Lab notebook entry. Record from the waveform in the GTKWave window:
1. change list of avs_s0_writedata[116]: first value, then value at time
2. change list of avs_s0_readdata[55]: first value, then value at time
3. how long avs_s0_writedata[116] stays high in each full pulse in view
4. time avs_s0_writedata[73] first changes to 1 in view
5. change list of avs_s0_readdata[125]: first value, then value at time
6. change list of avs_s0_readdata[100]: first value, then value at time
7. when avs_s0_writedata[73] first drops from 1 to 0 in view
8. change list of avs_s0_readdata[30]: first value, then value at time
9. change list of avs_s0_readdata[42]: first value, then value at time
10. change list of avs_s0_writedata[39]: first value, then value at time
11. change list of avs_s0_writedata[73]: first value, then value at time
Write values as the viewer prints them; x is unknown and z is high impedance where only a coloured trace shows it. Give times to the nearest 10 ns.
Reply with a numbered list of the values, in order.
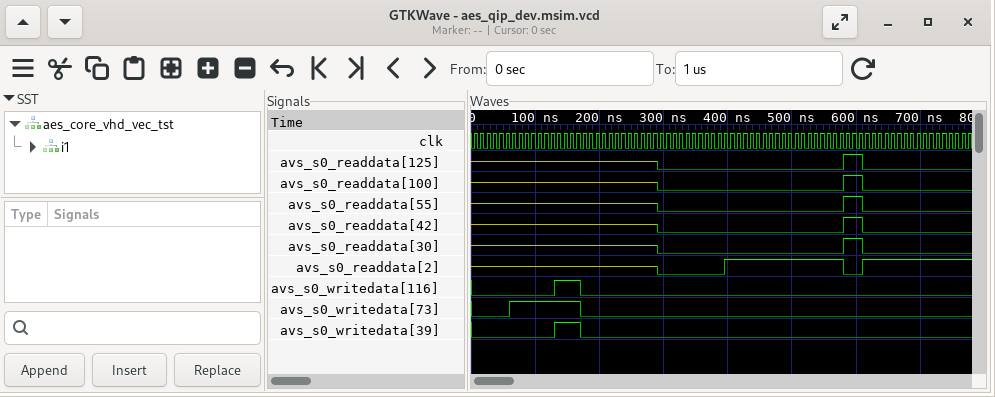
1. 0, 1 at 130 ns, 0 at 170 ns
2. z, 0 at 290 ns, 1 at 580 ns, 0 at 610 ns
3. 40 ns
4. 60 ns
5. z, 0 at 290 ns, 1 at 580 ns, 0 at 610 ns
6. z, 0 at 290 ns, 1 at 580 ns, 0 at 610 ns
7. 170 ns
8. z, 0 at 290 ns, 1 at 580 ns, 0 at 610 ns
9. z, 0 at 290 ns, 1 at 580 ns, 0 at 610 ns
10. 0, 1 at 130 ns, 0 at 170 ns
11. 0, 1 at 60 ns, 0 at 170 ns
